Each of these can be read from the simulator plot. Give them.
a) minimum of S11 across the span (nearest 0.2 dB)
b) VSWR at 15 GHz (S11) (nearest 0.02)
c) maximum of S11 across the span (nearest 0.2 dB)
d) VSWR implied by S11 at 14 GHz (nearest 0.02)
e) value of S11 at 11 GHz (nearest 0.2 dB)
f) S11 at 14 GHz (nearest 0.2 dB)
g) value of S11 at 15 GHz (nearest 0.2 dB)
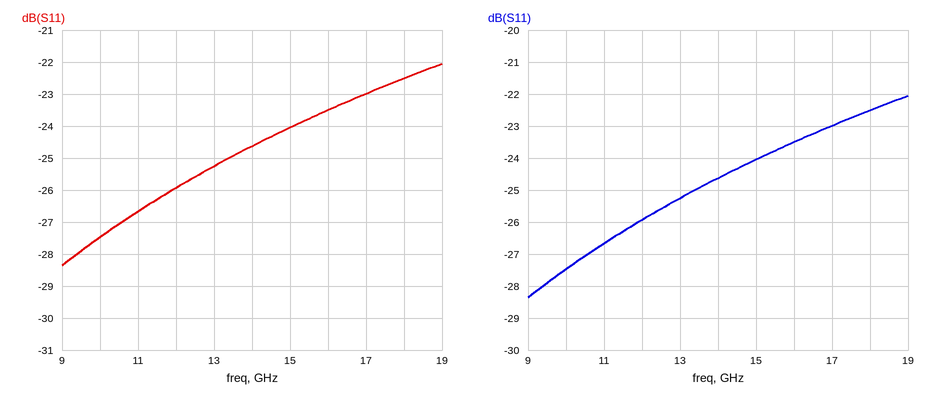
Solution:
-28.4 dB
1.14
-22.0 dB
1.12
-26.6 dB
-24.6 dB
-24.0 dB
